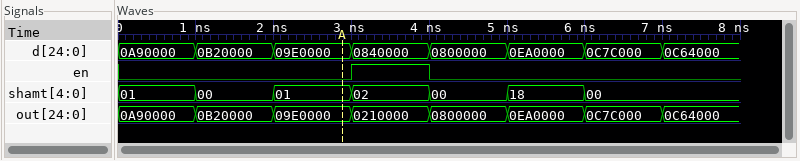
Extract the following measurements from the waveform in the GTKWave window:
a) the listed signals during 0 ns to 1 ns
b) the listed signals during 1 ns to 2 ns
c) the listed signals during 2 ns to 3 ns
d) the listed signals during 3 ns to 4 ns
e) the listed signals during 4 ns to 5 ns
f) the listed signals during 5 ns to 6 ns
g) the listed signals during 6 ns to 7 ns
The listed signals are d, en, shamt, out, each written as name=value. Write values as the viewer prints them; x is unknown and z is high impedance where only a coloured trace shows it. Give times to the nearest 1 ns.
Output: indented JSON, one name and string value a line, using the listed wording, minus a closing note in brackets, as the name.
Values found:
{
  "the listed signals during 0 ns to 1 ns": "d=0A90000, en=0, shamt=01, out=0A90000",
  "the listed signals during 1 ns to 2 ns": "d=0B20000, en=0, shamt=00, out=0B20000",
  "the listed signals during 2 ns to 3 ns": "d=09E0000, en=0, shamt=01, out=09E0000",
  "the listed signals during 3 ns to 4 ns": "d=0840000, en=1, shamt=02, out=0210000",
  "the listed signals during 4 ns to 5 ns": "d=0800000, en=0, shamt=00, out=0800000",
  "the listed signals during 5 ns to 6 ns": "d=0EA0000, en=0, shamt=18, out=0EA0000",
  "the listed signals during 6 ns to 7 ns": "d=0C7C000, en=0, shamt=00, out=0C7C000"
}
